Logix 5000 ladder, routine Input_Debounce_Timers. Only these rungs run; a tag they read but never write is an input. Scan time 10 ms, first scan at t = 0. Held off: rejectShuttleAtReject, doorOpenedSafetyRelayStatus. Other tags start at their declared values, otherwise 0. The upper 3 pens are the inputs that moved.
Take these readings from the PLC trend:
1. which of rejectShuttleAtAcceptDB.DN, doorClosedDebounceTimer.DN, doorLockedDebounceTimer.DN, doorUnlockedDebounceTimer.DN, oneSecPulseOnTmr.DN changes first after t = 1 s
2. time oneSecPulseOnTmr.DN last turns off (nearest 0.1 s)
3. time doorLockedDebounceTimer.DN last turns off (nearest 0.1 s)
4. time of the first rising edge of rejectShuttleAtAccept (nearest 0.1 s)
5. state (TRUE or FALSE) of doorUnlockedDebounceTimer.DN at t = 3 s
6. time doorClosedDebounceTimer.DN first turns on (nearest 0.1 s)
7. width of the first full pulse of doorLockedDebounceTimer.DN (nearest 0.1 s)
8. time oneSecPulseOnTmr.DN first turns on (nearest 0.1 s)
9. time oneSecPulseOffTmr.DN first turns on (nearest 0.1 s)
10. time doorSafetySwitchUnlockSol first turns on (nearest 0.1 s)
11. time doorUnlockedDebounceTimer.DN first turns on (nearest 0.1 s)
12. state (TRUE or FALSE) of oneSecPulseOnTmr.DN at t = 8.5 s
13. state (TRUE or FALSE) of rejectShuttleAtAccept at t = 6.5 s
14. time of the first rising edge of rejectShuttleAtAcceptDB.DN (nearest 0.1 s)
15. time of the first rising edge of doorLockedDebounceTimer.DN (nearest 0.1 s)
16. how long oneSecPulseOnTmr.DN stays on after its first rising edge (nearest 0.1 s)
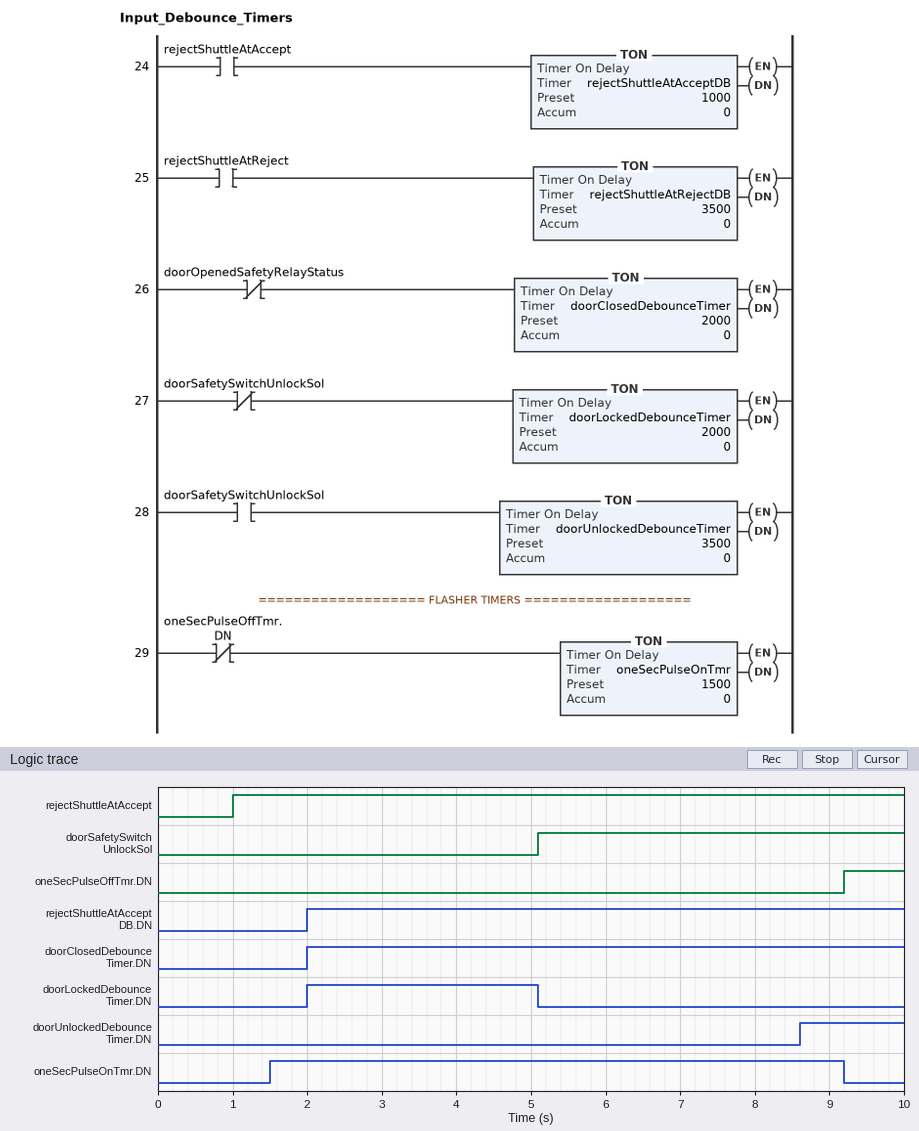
oneSecPulseOnTmr.DN
9.2 s
5.1 s
1.0 s
FALSE
2.0 s
3.1 s
1.5 s
9.2 s
5.1 s
8.6 s
TRUE
TRUE
2.0 s
2.0 s
7.7 s
